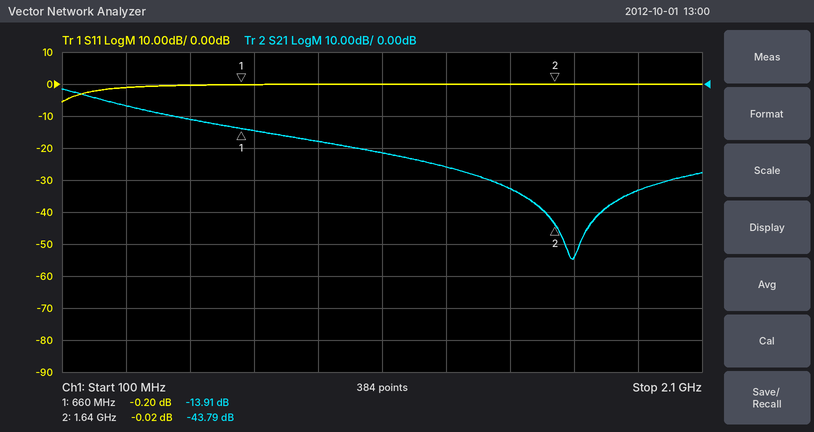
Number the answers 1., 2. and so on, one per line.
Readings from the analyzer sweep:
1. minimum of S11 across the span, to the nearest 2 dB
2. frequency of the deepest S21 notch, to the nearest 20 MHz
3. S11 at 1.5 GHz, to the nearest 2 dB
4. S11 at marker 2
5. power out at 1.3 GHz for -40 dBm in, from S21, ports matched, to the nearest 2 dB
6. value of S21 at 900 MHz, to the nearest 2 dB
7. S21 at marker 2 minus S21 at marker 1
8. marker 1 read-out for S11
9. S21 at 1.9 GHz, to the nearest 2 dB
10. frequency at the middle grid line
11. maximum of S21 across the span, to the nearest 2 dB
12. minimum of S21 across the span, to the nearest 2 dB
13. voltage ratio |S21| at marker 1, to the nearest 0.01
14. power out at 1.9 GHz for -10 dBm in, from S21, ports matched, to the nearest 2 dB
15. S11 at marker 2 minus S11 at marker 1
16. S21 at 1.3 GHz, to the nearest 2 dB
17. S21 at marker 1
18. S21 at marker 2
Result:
1. -6 dB
2. 1.70 GHz
3. 0 dB
4. -0.02 dB
5. -66 dBm
6. -18 dB
7. -29.88 dB
8. -0.20 dB
9. -34 dB
10. 1.1 GHz
11. -2 dB
12. -54 dB
13. 0.20
14. -44 dBm
15. 0.18 dB
16. -26 dB
17. -13.91 dB
18. -43.79 dB
